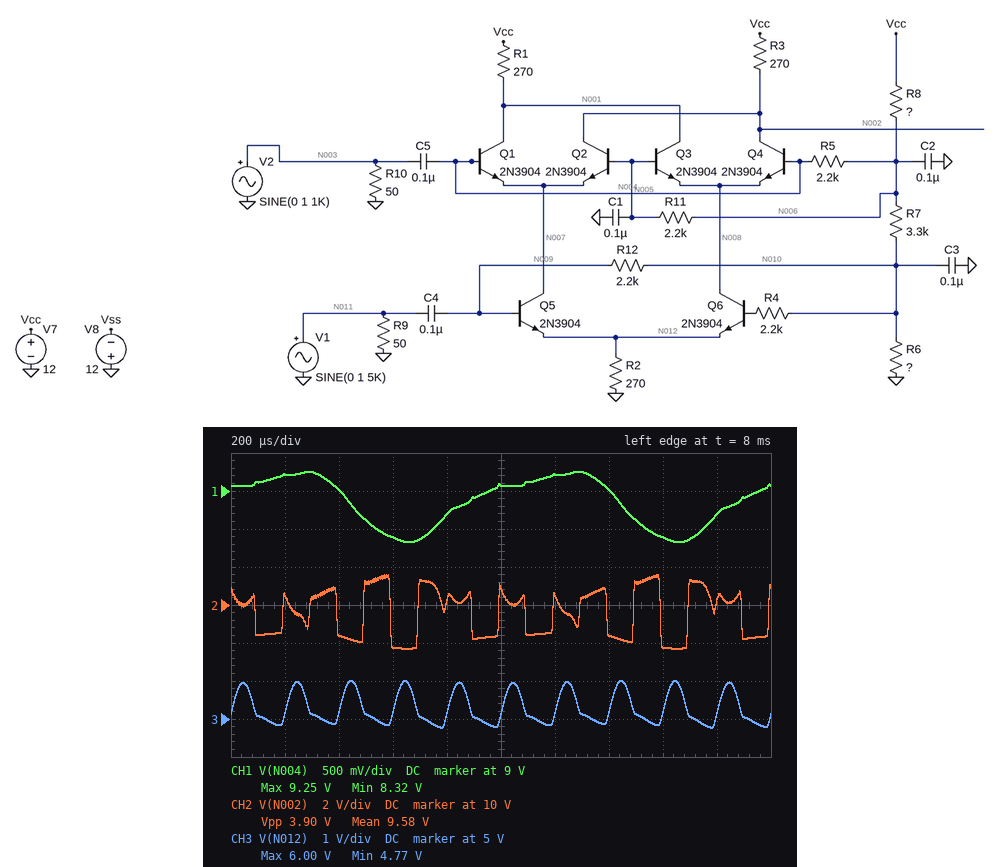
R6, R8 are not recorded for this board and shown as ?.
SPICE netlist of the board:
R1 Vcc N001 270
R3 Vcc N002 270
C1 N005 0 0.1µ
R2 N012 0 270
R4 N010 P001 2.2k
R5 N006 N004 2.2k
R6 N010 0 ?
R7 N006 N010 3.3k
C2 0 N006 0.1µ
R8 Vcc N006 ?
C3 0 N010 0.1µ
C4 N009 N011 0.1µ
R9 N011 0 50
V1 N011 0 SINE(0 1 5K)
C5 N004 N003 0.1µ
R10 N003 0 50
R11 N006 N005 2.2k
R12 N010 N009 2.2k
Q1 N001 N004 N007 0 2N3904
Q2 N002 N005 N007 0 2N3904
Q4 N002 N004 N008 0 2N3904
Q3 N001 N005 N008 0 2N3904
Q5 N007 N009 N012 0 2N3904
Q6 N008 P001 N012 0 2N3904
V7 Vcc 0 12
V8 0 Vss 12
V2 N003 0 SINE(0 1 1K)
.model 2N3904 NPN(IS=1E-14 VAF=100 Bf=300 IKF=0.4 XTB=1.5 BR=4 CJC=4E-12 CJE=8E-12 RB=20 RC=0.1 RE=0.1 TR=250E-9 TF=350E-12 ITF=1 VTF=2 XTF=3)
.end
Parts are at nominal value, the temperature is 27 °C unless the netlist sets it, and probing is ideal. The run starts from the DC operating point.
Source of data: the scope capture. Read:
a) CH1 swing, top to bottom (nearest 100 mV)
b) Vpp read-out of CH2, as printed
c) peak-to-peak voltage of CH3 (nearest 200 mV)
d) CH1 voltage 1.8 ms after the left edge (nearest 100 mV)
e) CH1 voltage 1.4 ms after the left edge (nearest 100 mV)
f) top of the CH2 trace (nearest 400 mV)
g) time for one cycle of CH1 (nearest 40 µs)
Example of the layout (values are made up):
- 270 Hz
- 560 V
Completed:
- 900 mV
- 3.90 V
- 1.2 V
- 8.7 V
- 9.0 V
- 11.6 V
- 1.00 ms
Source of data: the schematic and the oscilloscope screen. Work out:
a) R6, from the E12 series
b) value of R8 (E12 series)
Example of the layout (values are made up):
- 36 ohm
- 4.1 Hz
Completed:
- 5.6 kΩ
- 1.5 kΩ
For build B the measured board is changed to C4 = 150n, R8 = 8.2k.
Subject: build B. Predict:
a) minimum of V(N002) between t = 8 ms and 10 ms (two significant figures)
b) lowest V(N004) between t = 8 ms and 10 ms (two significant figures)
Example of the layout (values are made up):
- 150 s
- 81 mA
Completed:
- 8.1 V
- 5.2 V
